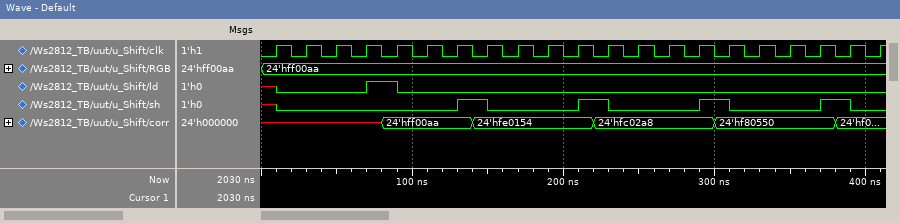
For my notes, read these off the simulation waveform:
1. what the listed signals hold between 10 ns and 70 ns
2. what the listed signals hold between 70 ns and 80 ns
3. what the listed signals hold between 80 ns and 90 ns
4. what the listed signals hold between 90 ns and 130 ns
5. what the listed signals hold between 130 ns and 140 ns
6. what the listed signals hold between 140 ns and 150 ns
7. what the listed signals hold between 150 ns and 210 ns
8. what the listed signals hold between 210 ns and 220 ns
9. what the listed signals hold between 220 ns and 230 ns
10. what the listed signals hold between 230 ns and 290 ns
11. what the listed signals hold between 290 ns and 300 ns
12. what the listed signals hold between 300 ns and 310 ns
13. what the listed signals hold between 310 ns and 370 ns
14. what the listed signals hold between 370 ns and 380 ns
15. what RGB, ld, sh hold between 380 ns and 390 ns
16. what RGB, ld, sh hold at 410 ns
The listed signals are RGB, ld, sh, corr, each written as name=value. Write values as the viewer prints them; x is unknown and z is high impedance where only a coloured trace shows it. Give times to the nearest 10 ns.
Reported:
RGB=24'hff00aa, ld=0, sh=0, corr=x
RGB=24'hff00aa, ld=1, sh=0, corr=x
RGB=24'hff00aa, ld=1, sh=0, corr=24'hff00aa
RGB=24'hff00aa, ld=0, sh=0, corr=24'hff00aa
RGB=24'hff00aa, ld=0, sh=1, corr=24'hff00aa
RGB=24'hff00aa, ld=0, sh=1, corr=24'hfe0154
RGB=24'hff00aa, ld=0, sh=0, corr=24'hfe0154
RGB=24'hff00aa, ld=0, sh=1, corr=24'hfe0154
RGB=24'hff00aa, ld=0, sh=1, corr=24'hfc02a8
RGB=24'hff00aa, ld=0, sh=0, corr=24'hfc02a8
RGB=24'hff00aa, ld=0, sh=1, corr=24'hfc02a8
RGB=24'hff00aa, ld=0, sh=1, corr=24'hf80550
RGB=24'hff00aa, ld=0, sh=0, corr=24'hf80550
RGB=24'hff00aa, ld=0, sh=1, corr=24'hf80550
RGB=24'hff00aa, ld=0, sh=1
RGB=24'hff00aa, ld=0, sh=0
